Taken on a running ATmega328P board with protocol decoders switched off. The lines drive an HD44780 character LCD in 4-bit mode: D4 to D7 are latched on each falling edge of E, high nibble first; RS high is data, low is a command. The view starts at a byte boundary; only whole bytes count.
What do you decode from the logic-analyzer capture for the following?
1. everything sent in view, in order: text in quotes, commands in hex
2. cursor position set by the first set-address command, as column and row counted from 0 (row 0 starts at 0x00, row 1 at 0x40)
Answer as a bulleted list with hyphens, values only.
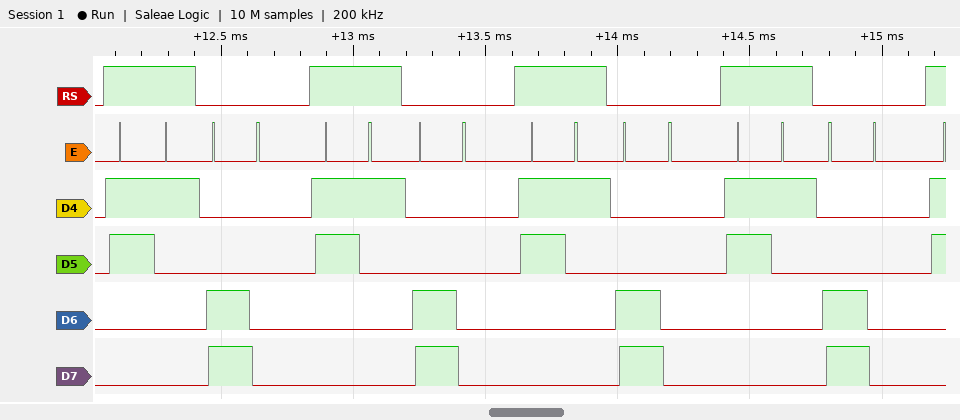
- "1" 0xC0 "1" 0xC0 "1" 0xC0 "1" 0xC0
- column 0, row 1
